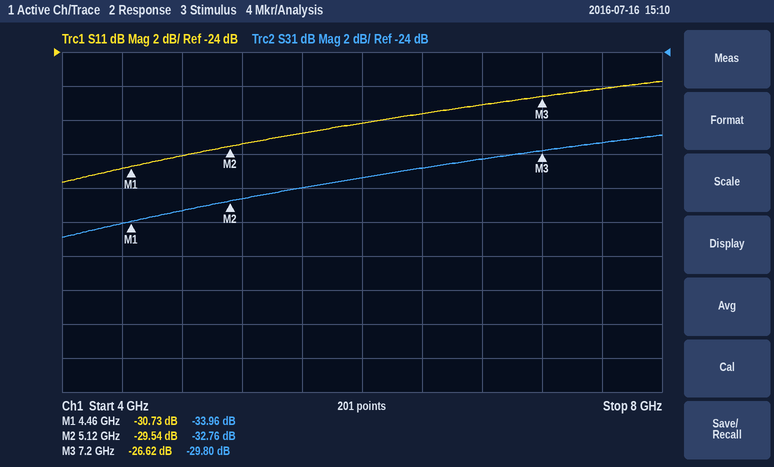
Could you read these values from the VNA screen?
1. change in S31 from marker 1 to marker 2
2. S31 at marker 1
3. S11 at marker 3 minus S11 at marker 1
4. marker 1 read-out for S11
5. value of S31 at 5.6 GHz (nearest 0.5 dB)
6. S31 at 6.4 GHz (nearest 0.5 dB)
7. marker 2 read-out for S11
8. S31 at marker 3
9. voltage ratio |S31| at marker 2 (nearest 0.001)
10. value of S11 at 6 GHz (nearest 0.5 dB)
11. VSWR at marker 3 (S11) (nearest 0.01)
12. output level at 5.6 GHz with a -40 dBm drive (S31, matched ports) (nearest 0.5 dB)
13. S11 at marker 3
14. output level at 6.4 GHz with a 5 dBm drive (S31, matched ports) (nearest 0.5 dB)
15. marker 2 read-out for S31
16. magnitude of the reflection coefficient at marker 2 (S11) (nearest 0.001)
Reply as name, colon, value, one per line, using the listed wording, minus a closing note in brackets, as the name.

change in S31 from marker 1 to marker 2: 1.20 dB
S31 at marker 1: -33.96 dB
S11 at marker 3 minus S11 at marker 1: 4.11 dB
marker 1 read-out for S11: -30.73 dB
value of S31 at 5.6 GHz: -32.0 dB
S31 at 6.4 GHz: -31.0 dB
marker 2 read-out for S11: -29.54 dB
S31 at marker 3: -29.80 dB
voltage ratio |S31| at marker 2: 0.023
value of S11 at 6 GHz: -28.0 dB
VSWR at marker 3 (S11): 1.10
output level at 5.6 GHz with a -40 dBm drive (S31, matched ports): -72.0 dBm
S11 at marker 3: -26.62 dB
output level at 6.4 GHz with a 5 dBm drive (S31, matched ports): -26.0 dBm
marker 2 read-out for S31: -32.76 dB
magnitude of the reflection coefficient at marker 2 (S11): 0.033
